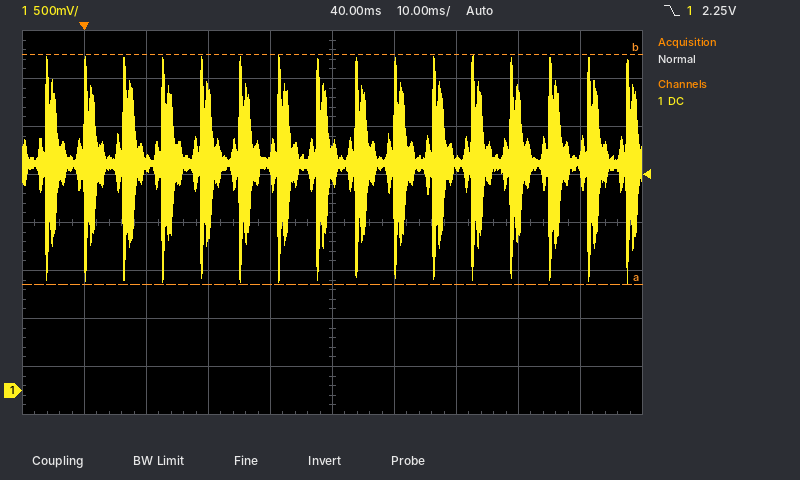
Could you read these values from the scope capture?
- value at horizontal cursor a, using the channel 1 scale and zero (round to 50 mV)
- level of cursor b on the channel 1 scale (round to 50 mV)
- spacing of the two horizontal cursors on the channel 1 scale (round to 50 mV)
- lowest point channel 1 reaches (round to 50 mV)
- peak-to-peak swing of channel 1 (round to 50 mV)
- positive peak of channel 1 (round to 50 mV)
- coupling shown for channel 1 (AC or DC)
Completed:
1.10 V
3.50 V
2.40 V
1.10 V
2.40 V
3.50 V
DC
